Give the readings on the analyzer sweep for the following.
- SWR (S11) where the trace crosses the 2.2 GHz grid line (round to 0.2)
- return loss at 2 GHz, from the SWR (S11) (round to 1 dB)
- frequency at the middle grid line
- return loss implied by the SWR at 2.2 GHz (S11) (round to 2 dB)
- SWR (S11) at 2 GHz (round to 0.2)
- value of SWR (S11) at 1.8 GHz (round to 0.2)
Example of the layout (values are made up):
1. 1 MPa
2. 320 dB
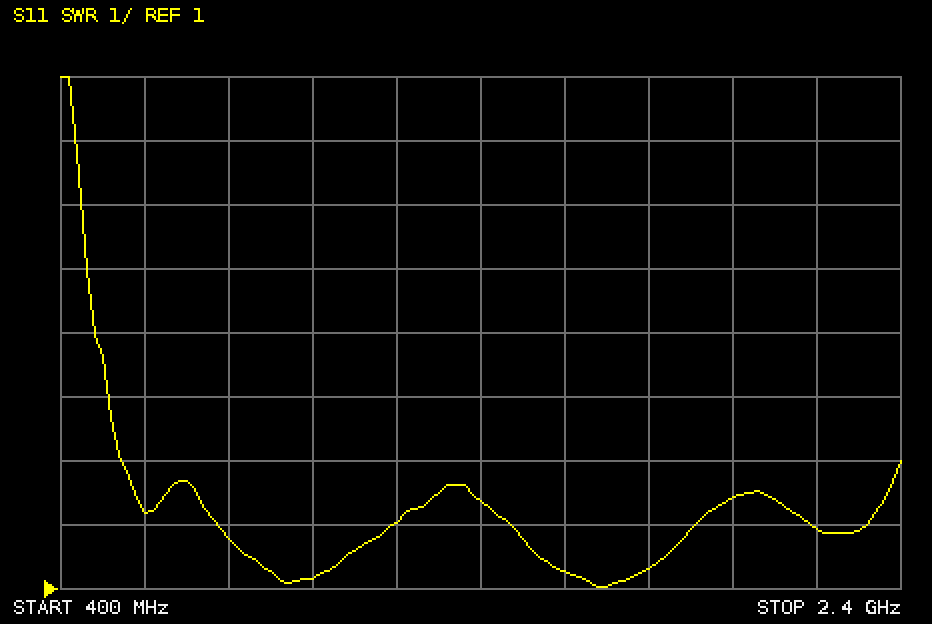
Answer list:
1. 2.0
2. 8 dB
3. 1.4 GHz
4. 10 dB
5. 2.4
6. 1.4
